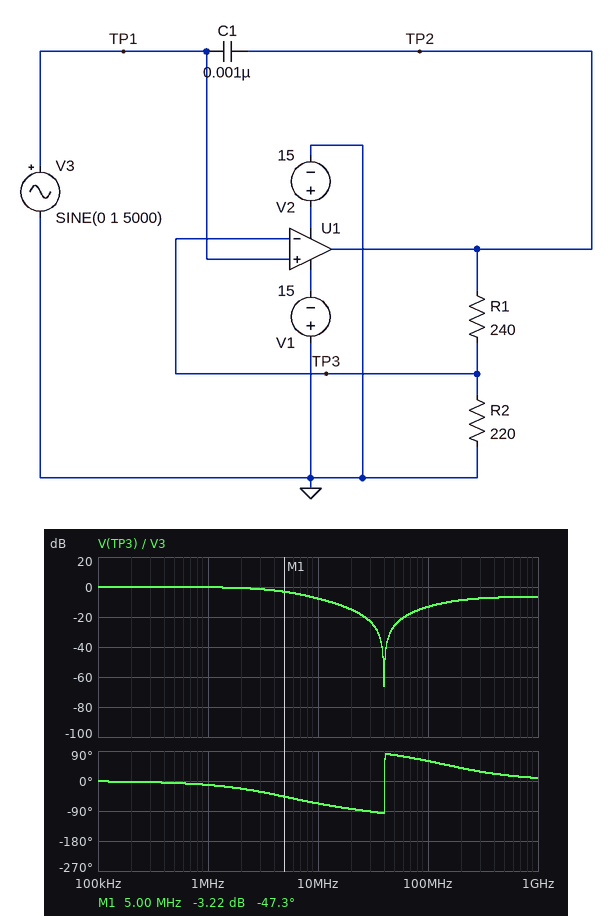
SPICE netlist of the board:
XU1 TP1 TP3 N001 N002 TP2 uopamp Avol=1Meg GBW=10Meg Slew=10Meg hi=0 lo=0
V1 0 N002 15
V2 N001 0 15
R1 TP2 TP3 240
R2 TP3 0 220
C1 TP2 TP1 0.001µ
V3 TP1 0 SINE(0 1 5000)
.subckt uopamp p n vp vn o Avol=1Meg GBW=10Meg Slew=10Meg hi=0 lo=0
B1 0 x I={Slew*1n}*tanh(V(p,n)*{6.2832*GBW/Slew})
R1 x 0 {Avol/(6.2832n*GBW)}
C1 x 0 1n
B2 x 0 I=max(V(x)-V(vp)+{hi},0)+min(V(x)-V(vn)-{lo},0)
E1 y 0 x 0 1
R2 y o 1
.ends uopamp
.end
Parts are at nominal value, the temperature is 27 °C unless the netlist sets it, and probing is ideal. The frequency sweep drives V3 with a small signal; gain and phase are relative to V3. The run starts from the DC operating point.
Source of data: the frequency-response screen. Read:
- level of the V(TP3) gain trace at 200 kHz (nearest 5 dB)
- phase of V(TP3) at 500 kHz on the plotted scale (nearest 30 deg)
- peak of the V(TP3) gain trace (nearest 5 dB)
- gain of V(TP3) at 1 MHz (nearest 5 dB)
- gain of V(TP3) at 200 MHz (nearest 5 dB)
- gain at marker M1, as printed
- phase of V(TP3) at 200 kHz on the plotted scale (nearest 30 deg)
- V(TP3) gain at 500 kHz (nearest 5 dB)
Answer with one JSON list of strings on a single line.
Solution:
["0 dB", "0 deg", "0 dB", "0 dB", "-10 dB", "-3.22 dB", "0 deg", "0 dB"]
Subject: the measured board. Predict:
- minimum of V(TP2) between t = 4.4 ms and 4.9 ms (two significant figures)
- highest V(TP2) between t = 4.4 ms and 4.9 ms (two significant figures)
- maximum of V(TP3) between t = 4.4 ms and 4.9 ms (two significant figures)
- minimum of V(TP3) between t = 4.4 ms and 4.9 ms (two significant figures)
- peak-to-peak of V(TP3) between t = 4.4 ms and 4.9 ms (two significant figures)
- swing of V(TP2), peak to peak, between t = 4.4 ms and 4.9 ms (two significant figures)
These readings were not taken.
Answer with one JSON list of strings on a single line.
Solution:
["-2.1 V", "2.1 V", "1.0 V", "-1.0 V", "2.0 V", "4.2 V"]
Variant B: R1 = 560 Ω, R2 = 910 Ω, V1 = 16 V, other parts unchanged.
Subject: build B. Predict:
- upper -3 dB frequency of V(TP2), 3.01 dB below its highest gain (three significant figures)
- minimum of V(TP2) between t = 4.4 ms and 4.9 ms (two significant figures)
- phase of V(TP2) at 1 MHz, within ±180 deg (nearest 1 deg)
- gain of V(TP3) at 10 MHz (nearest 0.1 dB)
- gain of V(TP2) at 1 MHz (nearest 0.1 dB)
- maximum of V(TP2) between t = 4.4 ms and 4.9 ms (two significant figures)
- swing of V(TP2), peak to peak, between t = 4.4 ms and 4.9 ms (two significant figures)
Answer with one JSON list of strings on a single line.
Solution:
["6.13 MHz", "-1.6 V", "-9 deg", "-5.9 dB", "4.1 dB", "1.6 V", "3.2 V"]
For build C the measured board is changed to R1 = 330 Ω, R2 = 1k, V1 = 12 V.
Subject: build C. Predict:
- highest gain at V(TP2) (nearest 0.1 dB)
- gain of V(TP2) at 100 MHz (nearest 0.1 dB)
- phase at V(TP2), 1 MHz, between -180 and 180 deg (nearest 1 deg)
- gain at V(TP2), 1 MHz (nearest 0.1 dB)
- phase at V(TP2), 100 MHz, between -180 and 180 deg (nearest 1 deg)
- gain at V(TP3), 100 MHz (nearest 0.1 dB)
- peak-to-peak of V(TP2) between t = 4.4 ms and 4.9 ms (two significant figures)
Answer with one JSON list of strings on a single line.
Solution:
["2.5 dB", "-6.7 dB", "-8 deg", "2.4 dB", "61 deg", "-9.2 dB", "2.7 V"]
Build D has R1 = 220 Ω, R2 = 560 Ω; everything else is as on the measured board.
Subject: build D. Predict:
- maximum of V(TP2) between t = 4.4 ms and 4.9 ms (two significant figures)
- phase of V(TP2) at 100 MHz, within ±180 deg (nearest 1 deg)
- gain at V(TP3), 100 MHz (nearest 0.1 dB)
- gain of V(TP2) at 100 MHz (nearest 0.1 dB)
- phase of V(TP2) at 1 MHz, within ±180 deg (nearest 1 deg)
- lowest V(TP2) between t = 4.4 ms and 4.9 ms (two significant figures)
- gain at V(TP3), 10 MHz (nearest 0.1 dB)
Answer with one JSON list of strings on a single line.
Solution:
["1.4 V", "61 deg", "-9.6 dB", "-6.7 dB", "-8 deg", "-1.4 V", "-5.0 dB"]
